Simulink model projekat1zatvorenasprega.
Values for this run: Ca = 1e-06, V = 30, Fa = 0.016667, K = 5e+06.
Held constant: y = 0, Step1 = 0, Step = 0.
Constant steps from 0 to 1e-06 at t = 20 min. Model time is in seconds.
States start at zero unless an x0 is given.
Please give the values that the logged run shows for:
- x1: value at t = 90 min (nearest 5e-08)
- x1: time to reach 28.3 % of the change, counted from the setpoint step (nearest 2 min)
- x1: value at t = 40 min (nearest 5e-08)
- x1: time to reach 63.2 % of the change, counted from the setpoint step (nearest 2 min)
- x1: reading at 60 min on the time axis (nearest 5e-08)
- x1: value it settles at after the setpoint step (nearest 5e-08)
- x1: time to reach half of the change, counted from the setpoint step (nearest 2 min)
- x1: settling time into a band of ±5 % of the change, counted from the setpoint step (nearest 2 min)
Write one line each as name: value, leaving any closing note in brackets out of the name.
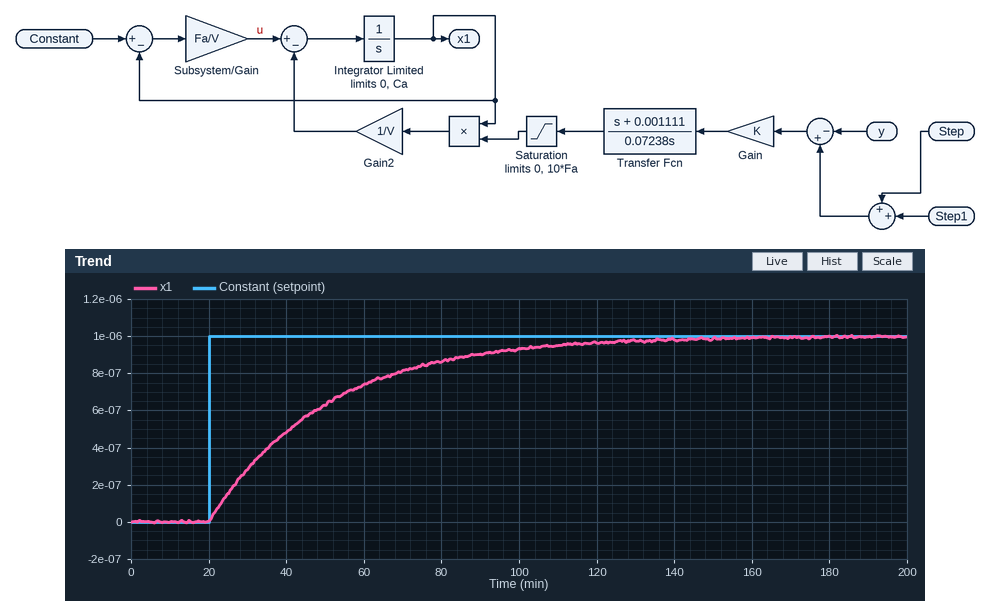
x1: value at t = 90 min: 0.00000090
x1: time to reach 28.3 % of the change, counted from the setpoint step: 10 min
x1: value at t = 40 min: 0.00000050
x1: time to reach 63.2 % of the change, counted from the setpoint step: 30 min
x1: reading at 60 min on the time axis: 0.00000075
x1: value it settles at after the setpoint step: 0.00000100
x1: time to reach half of the change, counted from the setpoint step: 20 min
x1: settling time into a band of ±5 % of the change, counted from the setpoint step: 90 min
